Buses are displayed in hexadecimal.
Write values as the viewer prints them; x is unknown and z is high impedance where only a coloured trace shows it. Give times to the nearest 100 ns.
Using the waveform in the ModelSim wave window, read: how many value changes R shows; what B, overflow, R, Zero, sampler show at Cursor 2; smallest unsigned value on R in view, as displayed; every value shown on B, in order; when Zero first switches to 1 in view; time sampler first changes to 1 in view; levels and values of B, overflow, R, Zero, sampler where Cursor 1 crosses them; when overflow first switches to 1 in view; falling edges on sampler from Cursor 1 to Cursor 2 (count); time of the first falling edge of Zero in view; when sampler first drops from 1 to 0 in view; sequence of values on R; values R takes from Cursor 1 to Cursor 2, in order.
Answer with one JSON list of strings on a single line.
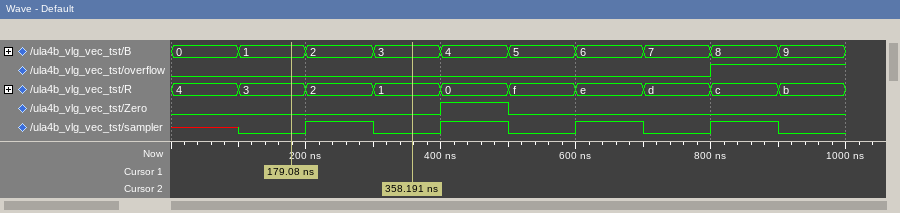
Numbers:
["9", "B=3, overflow=0, R=1, Zero=0, sampler=0", "0", "0, 1, 2, 3, 4, 5, 6, 7, 8, 9", "400 ns", "200 ns", "B=1, overflow=0, R=3, Zero=0, sampler=0", "800 ns", "1", "500 ns", "300 ns", "4, 3, 2, 1, 0, f, e, d, c, b", "3, 2, 1"]
